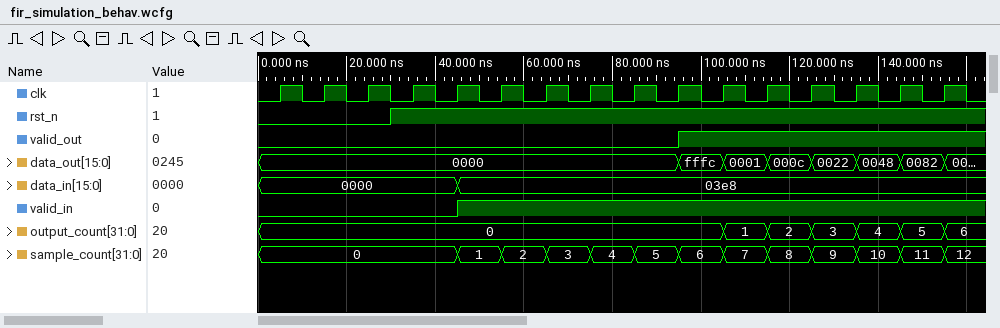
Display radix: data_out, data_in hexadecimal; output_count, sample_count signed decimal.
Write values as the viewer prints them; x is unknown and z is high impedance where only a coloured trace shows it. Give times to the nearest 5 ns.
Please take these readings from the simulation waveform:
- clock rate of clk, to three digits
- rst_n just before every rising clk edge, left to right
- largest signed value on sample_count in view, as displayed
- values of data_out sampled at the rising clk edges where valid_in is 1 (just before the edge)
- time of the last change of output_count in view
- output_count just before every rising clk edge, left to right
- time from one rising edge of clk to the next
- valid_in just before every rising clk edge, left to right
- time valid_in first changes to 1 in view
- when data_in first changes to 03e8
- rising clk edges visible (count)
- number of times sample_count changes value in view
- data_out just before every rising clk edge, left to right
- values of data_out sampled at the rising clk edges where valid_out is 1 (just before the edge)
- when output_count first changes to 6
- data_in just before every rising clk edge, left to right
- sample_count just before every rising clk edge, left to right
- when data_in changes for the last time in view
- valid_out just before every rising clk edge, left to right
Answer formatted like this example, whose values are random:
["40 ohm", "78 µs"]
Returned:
["100 MHz", "0 0 0 1 1 1 1 1 1 1 1 1 1 1 1 1", "12", "0000, 0000, 0000, 0000, 0000, fffc, 0001, 000c, 0022, 0048, 0082", "155 ns", "0, 0, 0, 0, 0, 0, 0, 0, 0, 0, 0, 1, 2, 3, 4, 5", "10 ns", "0 0 0 0 0 1 1 1 1 1 1 1 1 1 1 1", "45 ns", "45 ns", "16", "12", "0000, 0000, 0000, 0000, 0000, 0000, 0000, 0000, 0000, 0000, fffc, 0001, 000c, 0022, 0048, 0082", "fffc, 0001, 000c, 0022, 0048, 0082", "155 ns", "0000, 0000, 0000, 0000, 0000, 03e8, 03e8, 03e8, 03e8, 03e8, 03e8, 03e8, 03e8, 03e8, 03e8, 03e8", "0, 0, 0, 0, 0, 1, 2, 3, 4, 5, 6, 7, 8, 9, 10, 11", "45 ns", "0 0 0 0 0 0 0 0 0 0 1 1 1 1 1 1"]
